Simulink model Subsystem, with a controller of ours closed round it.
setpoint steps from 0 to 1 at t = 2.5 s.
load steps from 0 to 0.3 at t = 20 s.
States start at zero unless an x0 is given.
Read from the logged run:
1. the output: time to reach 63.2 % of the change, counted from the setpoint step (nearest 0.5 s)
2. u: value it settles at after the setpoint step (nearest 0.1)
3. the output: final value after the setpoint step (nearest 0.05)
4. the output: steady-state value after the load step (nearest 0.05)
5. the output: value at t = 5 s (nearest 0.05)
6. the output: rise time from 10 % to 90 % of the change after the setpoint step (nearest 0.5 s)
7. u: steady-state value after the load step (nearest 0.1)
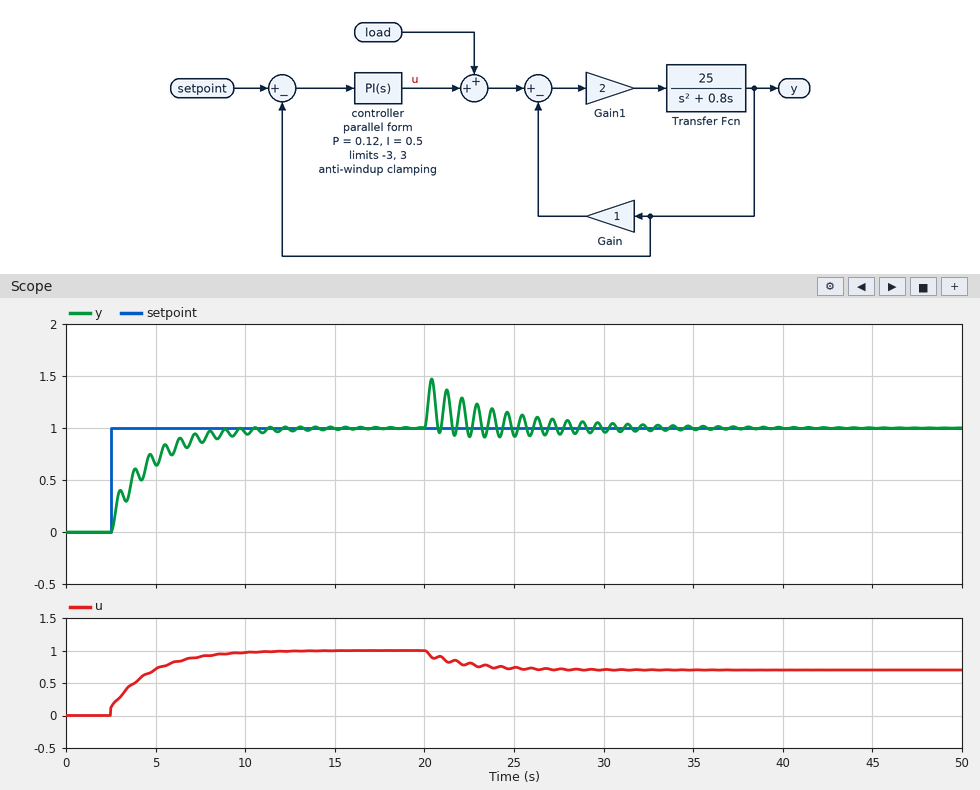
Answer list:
2.0 s
1.0
1.00
1.00
0.65
3.5 s
0.7
